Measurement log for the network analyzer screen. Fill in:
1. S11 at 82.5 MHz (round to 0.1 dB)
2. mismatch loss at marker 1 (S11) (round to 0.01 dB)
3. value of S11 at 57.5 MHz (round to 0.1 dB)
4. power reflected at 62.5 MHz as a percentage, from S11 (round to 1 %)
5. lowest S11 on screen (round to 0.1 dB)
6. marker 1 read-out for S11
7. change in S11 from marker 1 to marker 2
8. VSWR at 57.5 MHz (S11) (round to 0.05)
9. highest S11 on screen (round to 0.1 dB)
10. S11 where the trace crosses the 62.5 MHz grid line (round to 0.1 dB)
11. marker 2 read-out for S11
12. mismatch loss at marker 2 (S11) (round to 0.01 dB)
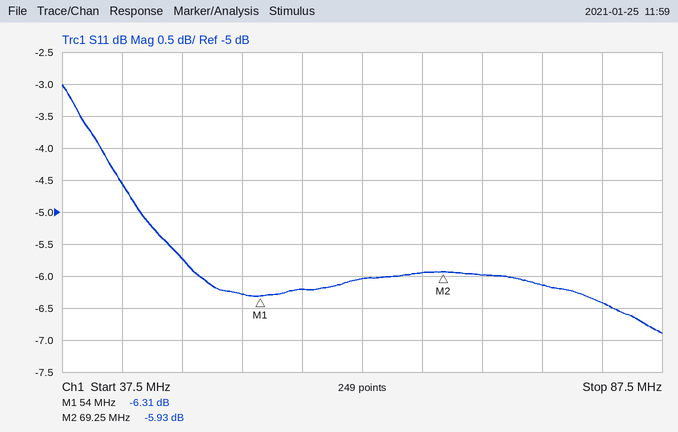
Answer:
-6.4 dB
1.16 dB
-6.2 dB
25 %
-6.9 dB
-6.31 dB
0.38 dB
2.90
-3.0 dB
-6.0 dB
-5.93 dB
1.28 dB
